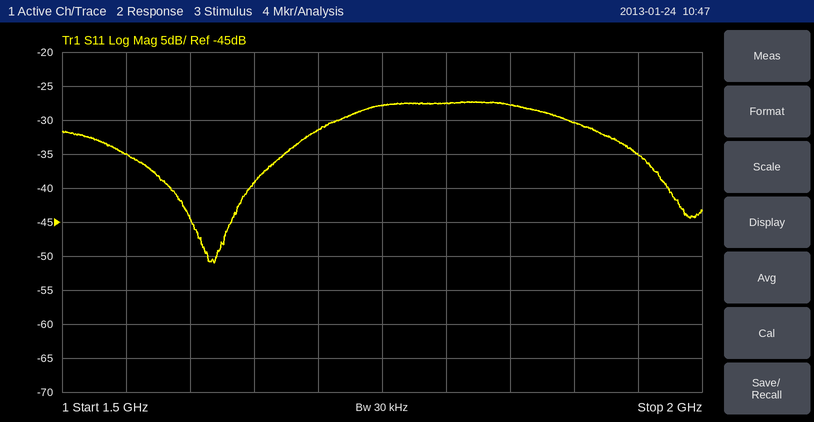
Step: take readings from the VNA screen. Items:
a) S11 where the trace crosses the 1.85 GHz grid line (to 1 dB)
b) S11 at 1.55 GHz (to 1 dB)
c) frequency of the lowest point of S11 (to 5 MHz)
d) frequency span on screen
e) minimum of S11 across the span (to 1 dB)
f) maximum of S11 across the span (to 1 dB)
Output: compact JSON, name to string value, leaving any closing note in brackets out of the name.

{"S11 where the trace crosses the 1.85 GHz grid line": "-28 dB", "S11 at 1.55 GHz": "-35 dB", "frequency of the lowest point of S11": "1.620 GHz", "frequency span on screen": "500 MHz", "minimum of S11 across the span": "-51 dB", "maximum of S11 across the span": "-27 dB"}
